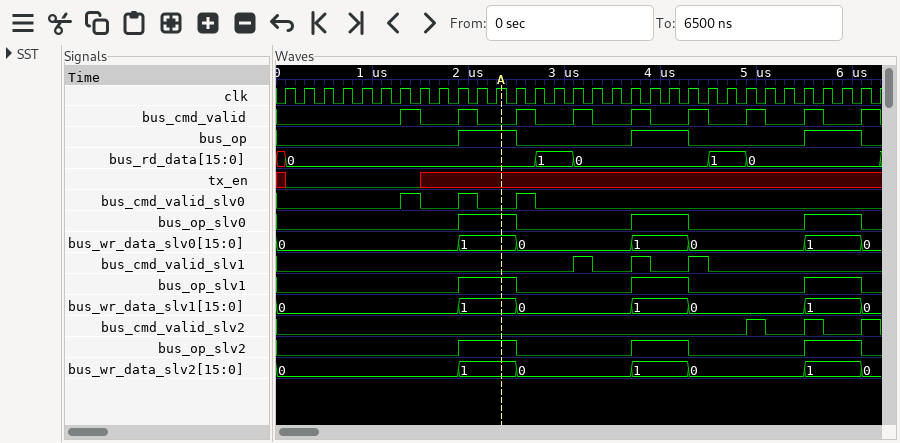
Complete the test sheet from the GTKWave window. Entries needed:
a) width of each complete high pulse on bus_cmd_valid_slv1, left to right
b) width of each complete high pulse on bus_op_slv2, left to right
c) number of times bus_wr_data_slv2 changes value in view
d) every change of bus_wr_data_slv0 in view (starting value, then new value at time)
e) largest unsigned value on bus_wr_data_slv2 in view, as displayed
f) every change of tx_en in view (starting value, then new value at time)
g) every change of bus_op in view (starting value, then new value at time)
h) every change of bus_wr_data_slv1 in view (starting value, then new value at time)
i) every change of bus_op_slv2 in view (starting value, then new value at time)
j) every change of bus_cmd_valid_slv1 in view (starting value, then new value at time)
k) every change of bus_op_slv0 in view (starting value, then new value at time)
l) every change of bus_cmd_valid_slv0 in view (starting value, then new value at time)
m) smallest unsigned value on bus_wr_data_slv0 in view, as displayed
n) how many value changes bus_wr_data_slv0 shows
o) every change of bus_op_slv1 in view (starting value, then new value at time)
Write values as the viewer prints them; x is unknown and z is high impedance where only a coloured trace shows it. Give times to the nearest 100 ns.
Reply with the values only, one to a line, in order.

200 ns, 200 ns, 200 ns
600 ns, 600 ns, 600 ns
6
0, 1 at 1900 ns, 0 at 2500 ns, 1 at 3700 ns, 0 at 4300 ns, 1 at 5500 ns, 0 at 6100 ns
1
x, 0 at 100 ns, x at 1500 ns
0, 1 at 1900 ns, 0 at 2500 ns, 1 at 3700 ns, 0 at 4300 ns, 1 at 5500 ns, 0 at 6100 ns
0, 1 at 1900 ns, 0 at 2500 ns, 1 at 3700 ns, 0 at 4300 ns, 1 at 5500 ns, 0 at 6100 ns
0, 1 at 1900 ns, 0 at 2500 ns, 1 at 3700 ns, 0 at 4300 ns, 1 at 5500 ns, 0 at 6100 ns
0, 1 at 3100 ns, 0 at 3300 ns, 1 at 3700 ns, 0 at 3900 ns, 1 at 4300 ns, 0 at 4500 ns
0, 1 at 1900 ns, 0 at 2500 ns, 1 at 3700 ns, 0 at 4300 ns, 1 at 5500 ns, 0 at 6100 ns
0, 1 at 1300 ns, 0 at 1500 ns, 1 at 1900 ns, 0 at 2100 ns, 1 at 2500 ns, 0 at 2700 ns
0
6
0, 1 at 1900 ns, 0 at 2500 ns, 1 at 3700 ns, 0 at 4300 ns, 1 at 5500 ns, 0 at 6100 ns
